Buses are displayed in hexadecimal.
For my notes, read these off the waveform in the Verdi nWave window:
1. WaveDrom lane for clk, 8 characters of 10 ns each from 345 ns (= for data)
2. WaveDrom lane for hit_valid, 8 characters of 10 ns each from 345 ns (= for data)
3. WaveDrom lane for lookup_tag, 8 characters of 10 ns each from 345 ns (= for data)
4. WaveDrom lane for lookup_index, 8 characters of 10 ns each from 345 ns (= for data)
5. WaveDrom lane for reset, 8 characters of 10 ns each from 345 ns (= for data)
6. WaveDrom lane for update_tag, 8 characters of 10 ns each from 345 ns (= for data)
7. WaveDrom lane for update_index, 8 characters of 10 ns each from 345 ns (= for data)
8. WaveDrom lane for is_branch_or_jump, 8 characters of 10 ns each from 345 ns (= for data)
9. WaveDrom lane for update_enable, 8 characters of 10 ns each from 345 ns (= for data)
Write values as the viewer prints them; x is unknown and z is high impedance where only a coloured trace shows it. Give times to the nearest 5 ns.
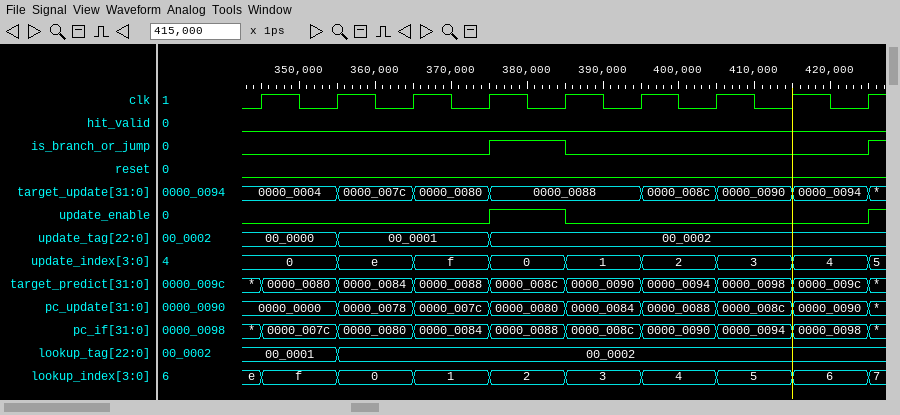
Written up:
{name: 'clk', wave: 'p.......'}
{name: 'hit_valid', wave: '0.......'}
{name: 'lookup_tag', wave: '==......', data: '00_0001 00_0002'}
{name: 'lookup_index', wave: '========', data: 'f 0 1 2 3 4 5 6'}
{name: 'reset', wave: '0.......'}
{name: 'update_tag', wave: '==.=....', data: '00_0000 00_0001 00_0002'}
{name: 'update_index', wave: '========', data: '0 e f 0 1 2 3 4'}
{name: 'is_branch_or_jump', wave: '0..10...'}
{name: 'update_enable', wave: '0..10...'}
